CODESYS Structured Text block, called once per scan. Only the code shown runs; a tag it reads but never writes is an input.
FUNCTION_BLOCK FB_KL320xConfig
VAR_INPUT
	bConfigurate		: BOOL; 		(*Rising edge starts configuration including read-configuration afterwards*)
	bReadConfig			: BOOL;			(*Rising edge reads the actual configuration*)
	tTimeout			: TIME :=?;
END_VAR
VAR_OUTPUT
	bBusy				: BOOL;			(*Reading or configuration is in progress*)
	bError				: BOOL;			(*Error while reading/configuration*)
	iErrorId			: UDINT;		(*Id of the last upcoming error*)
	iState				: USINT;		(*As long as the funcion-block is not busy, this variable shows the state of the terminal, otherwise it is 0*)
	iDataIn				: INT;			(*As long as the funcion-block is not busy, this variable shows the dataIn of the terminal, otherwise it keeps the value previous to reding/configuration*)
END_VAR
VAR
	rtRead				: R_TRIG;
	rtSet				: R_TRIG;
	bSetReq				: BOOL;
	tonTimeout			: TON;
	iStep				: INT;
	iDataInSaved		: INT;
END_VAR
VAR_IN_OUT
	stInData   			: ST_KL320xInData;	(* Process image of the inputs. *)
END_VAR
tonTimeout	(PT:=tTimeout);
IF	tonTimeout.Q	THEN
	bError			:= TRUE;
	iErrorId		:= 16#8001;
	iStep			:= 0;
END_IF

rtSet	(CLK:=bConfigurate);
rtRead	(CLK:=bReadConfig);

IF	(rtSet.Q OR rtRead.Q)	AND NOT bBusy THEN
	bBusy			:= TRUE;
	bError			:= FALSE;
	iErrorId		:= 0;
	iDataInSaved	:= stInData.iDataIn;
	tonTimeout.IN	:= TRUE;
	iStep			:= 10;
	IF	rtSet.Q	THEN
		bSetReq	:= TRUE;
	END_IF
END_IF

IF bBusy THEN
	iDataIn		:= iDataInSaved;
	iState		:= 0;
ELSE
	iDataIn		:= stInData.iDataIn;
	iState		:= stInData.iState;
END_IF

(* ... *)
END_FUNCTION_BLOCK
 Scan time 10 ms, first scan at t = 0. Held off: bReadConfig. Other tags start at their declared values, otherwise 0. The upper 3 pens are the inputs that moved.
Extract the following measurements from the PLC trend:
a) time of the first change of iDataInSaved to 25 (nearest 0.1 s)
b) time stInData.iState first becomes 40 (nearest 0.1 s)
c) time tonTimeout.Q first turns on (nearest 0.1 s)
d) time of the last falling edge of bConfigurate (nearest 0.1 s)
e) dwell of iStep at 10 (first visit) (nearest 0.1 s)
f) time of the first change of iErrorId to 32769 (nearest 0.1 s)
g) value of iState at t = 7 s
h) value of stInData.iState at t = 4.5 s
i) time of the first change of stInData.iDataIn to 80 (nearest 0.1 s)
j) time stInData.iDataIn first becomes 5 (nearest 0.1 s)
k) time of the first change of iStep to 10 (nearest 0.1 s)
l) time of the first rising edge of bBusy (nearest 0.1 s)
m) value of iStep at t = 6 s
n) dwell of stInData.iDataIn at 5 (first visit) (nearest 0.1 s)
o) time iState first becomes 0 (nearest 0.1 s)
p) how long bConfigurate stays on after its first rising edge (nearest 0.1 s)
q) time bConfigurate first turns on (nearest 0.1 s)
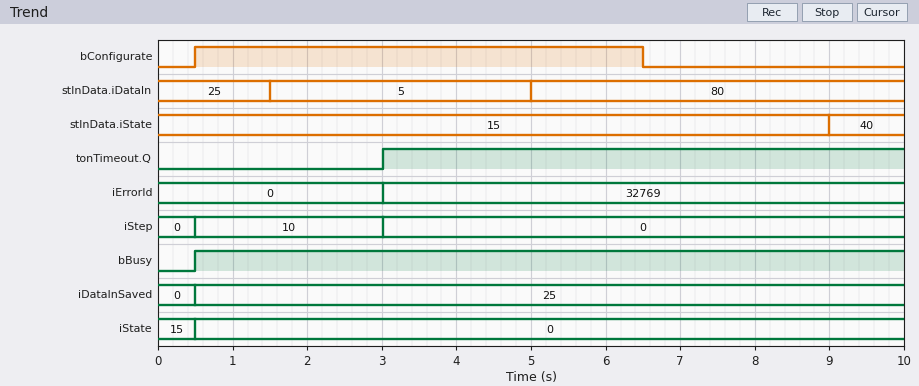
0.5 s
9.0 s
3.0 s
6.5 s
2.5 s
3.0 s
0
15
5.0 s
1.5 s
0.5 s
0.5 s
0
3.5 s
0.5 s
6.0 s
0.5 s
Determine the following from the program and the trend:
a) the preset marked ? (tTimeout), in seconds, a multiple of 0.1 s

2.5 s
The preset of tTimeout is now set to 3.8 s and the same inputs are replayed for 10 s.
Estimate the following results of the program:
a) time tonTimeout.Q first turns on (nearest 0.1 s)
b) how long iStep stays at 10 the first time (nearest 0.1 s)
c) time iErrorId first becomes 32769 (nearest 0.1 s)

4.3 s
3.8 s
4.3 s
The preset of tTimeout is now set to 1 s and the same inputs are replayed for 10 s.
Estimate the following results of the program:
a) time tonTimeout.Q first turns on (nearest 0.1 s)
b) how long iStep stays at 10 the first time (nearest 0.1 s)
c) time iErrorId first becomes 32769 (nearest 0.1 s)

1.5 s
1.0 s
1.5 s
